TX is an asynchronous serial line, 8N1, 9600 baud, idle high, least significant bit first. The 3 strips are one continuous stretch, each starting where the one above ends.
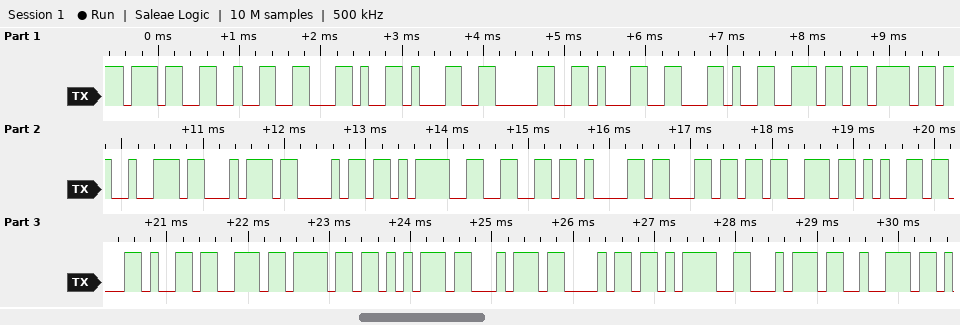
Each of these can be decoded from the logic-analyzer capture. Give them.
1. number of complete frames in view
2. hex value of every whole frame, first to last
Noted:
27
37 32 2C 31 30 31 2C 6E 6F 72 74 68 3D 66 61 6C 73 65 2C 73 6F 75 74 68 3D 74 72
